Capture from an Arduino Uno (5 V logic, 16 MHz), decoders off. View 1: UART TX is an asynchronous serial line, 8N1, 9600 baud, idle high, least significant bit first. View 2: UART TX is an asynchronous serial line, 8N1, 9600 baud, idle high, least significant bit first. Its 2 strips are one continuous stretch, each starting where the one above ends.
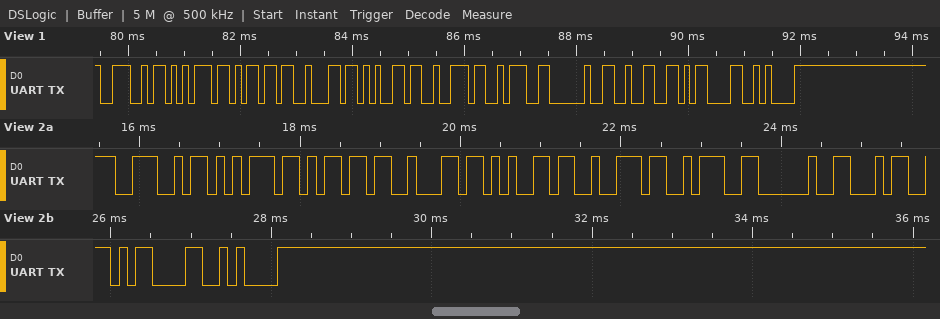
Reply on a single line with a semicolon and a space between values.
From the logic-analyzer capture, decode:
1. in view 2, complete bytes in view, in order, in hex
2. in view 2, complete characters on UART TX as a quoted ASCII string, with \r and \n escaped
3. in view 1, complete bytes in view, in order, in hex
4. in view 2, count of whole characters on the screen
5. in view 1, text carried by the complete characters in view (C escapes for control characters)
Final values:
4E 75 6D 62 65 72 3A 20 34 0D 0A; "Number: 4\r\n"; 4E 75 6D 62 65 72 3A 20 32 0D 0A; 11; "Number: 2\r\n"
